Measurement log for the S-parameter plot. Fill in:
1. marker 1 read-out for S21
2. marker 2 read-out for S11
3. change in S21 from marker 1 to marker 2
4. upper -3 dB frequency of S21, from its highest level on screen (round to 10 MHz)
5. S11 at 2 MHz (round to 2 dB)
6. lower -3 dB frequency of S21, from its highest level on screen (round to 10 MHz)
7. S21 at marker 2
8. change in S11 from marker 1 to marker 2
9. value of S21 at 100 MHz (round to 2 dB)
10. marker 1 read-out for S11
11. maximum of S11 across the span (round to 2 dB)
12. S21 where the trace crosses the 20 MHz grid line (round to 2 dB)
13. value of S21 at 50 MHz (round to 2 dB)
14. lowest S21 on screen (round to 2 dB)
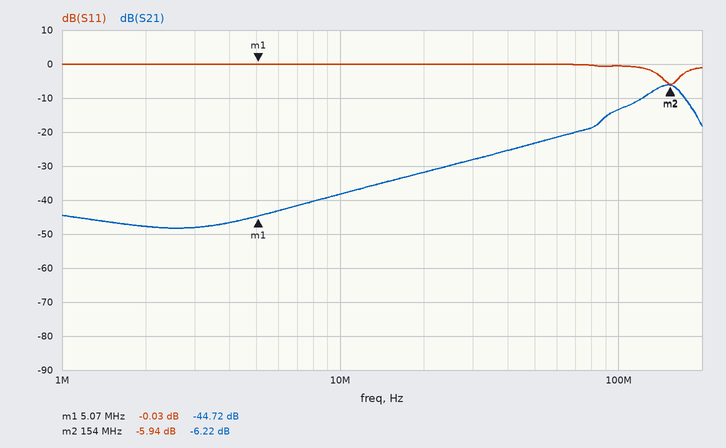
-44.72 dB
-5.94 dB
38.50 dB
170 MHz
0 dB
130 MHz
-6.22 dB
-5.91 dB
-14 dB
-0.03 dB
0 dB
-32 dB
-24 dB
-48 dB
